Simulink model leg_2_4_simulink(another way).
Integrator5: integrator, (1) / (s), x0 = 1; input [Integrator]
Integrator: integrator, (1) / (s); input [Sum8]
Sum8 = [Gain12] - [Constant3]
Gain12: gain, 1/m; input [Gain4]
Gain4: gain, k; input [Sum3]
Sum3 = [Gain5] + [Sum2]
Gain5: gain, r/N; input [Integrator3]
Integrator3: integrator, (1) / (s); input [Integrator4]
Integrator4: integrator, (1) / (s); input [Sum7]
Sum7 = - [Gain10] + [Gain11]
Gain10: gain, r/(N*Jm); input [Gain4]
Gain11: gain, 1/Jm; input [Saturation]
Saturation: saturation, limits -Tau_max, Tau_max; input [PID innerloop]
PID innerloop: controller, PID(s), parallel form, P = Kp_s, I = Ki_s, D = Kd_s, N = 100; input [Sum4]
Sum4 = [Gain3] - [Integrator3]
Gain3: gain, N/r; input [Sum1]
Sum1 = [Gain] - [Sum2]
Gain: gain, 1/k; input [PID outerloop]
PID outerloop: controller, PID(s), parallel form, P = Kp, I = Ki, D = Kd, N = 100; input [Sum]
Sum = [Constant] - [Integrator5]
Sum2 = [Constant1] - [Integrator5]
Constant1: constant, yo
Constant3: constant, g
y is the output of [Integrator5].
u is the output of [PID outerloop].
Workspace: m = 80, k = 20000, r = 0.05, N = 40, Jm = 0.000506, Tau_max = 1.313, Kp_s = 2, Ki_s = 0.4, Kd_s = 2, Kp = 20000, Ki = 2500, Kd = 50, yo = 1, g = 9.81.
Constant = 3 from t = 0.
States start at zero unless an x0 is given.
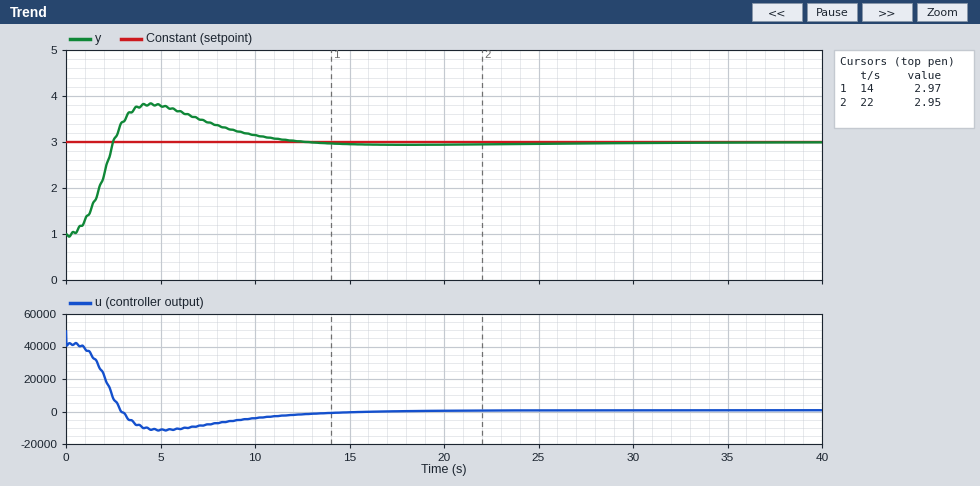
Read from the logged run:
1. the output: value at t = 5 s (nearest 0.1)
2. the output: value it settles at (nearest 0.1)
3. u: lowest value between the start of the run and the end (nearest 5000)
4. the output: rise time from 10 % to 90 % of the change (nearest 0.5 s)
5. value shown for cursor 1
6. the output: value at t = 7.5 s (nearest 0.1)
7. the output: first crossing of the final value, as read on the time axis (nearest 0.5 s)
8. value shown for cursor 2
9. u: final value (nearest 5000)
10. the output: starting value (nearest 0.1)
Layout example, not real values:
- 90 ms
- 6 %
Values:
- 3.8
- 3.0
- -10000
- 1.5 s
- 2.97
- 3.4
- 2.5 s
- 2.95
- 0
- 1.0
